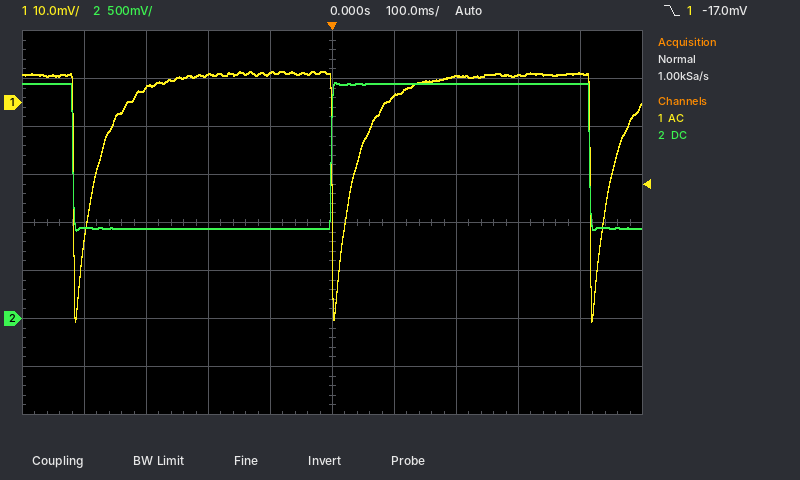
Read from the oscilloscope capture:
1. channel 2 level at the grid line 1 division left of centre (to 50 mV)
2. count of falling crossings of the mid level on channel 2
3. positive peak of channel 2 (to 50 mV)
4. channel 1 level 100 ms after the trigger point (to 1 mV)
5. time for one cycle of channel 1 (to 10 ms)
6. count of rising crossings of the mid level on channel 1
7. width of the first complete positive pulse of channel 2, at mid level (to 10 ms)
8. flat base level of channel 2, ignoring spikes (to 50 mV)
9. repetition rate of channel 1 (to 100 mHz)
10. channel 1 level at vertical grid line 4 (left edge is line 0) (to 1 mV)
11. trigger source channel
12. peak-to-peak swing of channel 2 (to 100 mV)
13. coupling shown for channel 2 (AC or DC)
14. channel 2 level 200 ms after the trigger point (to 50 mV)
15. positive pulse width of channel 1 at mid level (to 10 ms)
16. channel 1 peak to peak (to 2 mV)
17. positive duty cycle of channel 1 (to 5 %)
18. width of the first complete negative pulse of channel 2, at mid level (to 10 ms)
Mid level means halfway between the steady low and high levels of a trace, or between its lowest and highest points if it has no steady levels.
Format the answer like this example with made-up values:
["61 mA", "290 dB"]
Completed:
["950 mV", "2", "2.45 V", "1 mV", "420 ms", "3", "420 ms", "950 mV", "2.4 Hz", "6 mV", "channel 1", "1.50 V", "DC", "2.45 V", "390 ms", "52 mV", "95 %", "420 ms"]
